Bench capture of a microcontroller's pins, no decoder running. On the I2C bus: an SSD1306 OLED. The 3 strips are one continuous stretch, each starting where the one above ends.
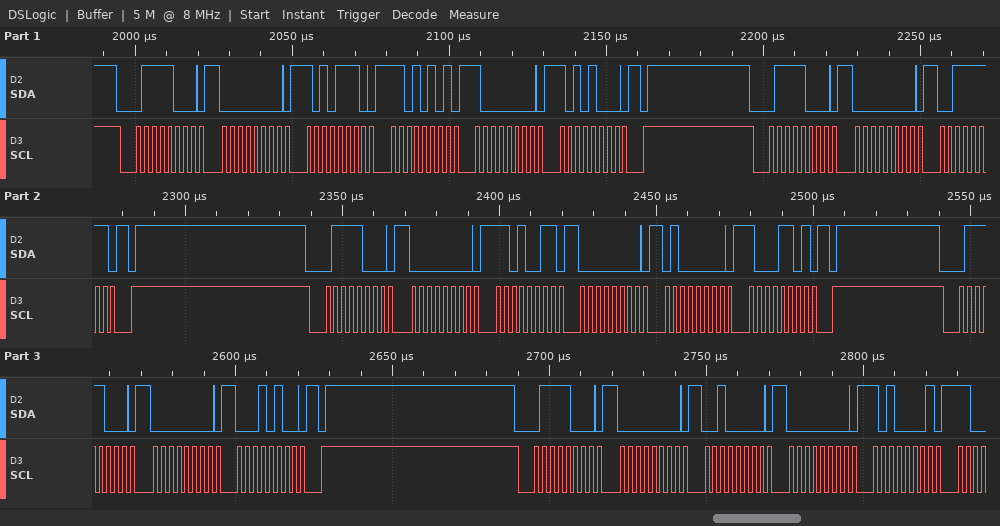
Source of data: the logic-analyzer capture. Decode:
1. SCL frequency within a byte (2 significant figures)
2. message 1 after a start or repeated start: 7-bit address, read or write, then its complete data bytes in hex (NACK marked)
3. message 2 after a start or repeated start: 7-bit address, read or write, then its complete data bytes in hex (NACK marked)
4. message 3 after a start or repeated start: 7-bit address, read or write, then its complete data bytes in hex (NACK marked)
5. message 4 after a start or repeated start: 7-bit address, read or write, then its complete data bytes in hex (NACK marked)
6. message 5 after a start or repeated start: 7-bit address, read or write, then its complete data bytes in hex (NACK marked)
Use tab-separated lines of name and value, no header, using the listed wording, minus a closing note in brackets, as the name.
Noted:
SCL frequency within a byte	400 kHz
message 1 after a start or repeated start: 7-bit address, read or write, then its complete data bytes in hex	0x3C write: 00 AE D5 80 A8
message 2 after a start or repeated start: 7-bit address, read or write, then its complete data bytes in hex	0x3C write: 00 3F
message 3 after a start or repeated start: 7-bit address, read or write, then its complete data bytes in hex	0x3C write: 00 D3 00 40 8D
message 4 after a start or repeated start: 7-bit address, read or write, then its complete data bytes in hex	0x3C write: 00 14
message 5 after a start or repeated start: 7-bit address, read or write, then its complete data bytes in hex	0x3C write: 00 20 00 A1
